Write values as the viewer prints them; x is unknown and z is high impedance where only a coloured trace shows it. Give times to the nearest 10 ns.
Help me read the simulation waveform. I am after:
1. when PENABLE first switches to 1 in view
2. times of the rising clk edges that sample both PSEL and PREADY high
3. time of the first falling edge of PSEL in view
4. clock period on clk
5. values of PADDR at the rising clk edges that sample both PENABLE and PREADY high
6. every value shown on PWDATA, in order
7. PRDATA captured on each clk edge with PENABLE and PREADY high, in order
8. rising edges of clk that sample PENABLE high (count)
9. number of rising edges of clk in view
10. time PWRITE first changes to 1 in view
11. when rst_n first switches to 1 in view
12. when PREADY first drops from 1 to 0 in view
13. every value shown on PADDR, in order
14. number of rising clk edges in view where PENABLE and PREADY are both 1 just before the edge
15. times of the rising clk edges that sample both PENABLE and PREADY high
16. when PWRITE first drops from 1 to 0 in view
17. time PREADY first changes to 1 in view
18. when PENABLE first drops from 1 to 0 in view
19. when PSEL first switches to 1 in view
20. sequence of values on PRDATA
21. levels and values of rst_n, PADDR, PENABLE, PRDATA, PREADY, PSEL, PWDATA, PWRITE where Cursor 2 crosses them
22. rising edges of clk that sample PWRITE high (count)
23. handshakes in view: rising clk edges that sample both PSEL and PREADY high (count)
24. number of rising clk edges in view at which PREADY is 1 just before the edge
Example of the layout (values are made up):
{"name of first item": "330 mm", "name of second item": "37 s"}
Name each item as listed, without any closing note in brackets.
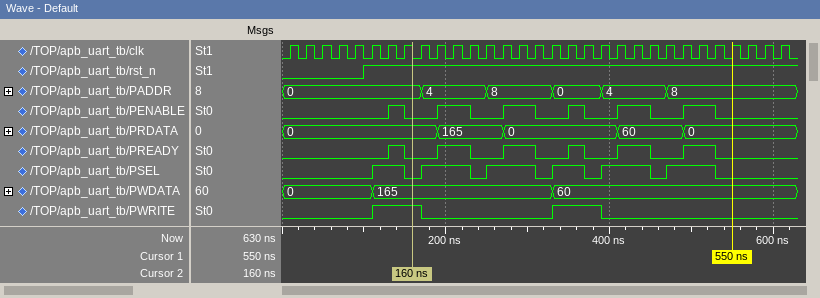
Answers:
{"when PENABLE first switches to 1 in view": "130 ns", "times of the rising clk edges that sample both PSEL and PREADY high": "150 ns, 210 ns, 230 ns, 290 ns, 310 ns, 370 ns, 430 ns, 450 ns, 510 ns, 530 ns", "time of the first falling edge of PSEL in view": "150 ns", "clock period on clk": "20 ns", "values of PADDR at the rising clk edges that sample both PENABLE and PREADY high": "0, 4, 4, 8, 8, 0, 4, 4, 8, 8", "every value shown on PWDATA, in order": "0, 165, 60", "PRDATA captured on each clk edge with PENABLE and PREADY high, in order": "0, 165, 165, 0, 0, 0, 60, 60, 0, 0", "rising edges of clk that sample PENABLE high": "10", "number of rising edges of clk in view": "31", "time PWRITE first changes to 1 in view": "110 ns", "when rst_n first switches to 1 in view": "100 ns", "when PREADY first drops from 1 to 0 in view": "150 ns", "every value shown on PADDR, in order": "0, 4, 8, 0, 4, 8", "number of rising clk edges in view where PENABLE and PREADY are both 1 just before the edge": "10", "times of the rising clk edges that sample both PENABLE and PREADY high": "150 ns, 210 ns, 230 ns, 290 ns, 310 ns, 370 ns, 430 ns, 450 ns, 510 ns, 530 ns", "when PWRITE first drops from 1 to 0 in view": "170 ns", "time PREADY first changes to 1 in view": "130 ns", "when PENABLE first drops from 1 to 0 in view": "150 ns", "when PSEL first switches to 1 in view": "110 ns", "sequence of values on PRDATA": "0, 165, 0, 60, 0", "levels and values of rst_n, PADDR, PENABLE, PRDATA, PREADY, PSEL, PWDATA, PWRITE where Cursor 2 crosses them": "rst_n=1, PADDR=0, PENABLE=0, PRDATA=0, PREADY=0, PSEL=0, PWDATA=165, PWRITE=1", "rising edges of clk that sample PWRITE high": "6", "handshakes in view: rising clk edges that sample both PSEL and PREADY high": "10", "number of rising clk edges in view at which PREADY is 1 just before the edge": "10"}
